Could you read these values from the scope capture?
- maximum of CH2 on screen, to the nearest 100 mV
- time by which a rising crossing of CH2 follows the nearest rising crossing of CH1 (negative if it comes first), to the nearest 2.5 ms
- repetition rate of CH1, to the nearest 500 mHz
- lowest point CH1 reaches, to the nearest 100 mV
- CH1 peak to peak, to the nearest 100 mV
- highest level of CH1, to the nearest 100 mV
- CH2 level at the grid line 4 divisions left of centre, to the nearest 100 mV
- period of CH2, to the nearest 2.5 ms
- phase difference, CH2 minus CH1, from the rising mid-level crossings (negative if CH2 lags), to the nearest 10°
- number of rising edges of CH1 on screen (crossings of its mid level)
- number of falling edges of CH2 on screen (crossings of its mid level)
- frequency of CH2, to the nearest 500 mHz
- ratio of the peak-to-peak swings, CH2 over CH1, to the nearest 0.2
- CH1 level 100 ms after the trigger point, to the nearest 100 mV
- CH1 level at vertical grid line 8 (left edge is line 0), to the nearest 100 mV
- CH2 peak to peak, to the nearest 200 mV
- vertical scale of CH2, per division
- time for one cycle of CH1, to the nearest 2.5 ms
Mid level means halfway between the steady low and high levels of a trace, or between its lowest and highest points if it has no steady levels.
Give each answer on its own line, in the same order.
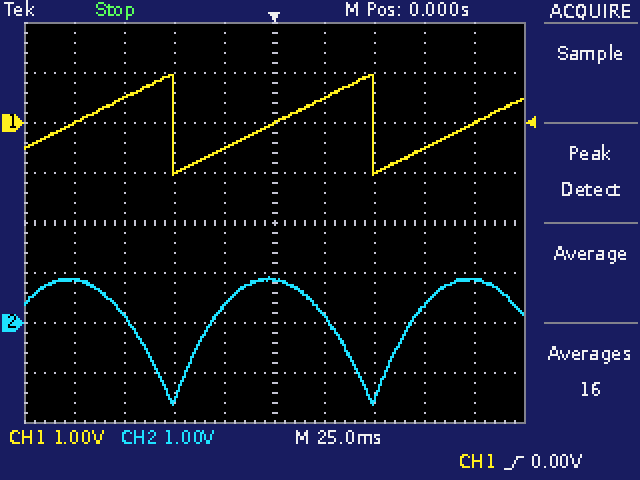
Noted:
900 mV
-35.0 ms
10.0 Hz
-1.0 V
2.0 V
1.0 V
900 mV
100.0 ms
+130°
3
2
10.0 Hz
1.2
0.0 V
-500 mV
2.6 V
1 V
100.0 ms
